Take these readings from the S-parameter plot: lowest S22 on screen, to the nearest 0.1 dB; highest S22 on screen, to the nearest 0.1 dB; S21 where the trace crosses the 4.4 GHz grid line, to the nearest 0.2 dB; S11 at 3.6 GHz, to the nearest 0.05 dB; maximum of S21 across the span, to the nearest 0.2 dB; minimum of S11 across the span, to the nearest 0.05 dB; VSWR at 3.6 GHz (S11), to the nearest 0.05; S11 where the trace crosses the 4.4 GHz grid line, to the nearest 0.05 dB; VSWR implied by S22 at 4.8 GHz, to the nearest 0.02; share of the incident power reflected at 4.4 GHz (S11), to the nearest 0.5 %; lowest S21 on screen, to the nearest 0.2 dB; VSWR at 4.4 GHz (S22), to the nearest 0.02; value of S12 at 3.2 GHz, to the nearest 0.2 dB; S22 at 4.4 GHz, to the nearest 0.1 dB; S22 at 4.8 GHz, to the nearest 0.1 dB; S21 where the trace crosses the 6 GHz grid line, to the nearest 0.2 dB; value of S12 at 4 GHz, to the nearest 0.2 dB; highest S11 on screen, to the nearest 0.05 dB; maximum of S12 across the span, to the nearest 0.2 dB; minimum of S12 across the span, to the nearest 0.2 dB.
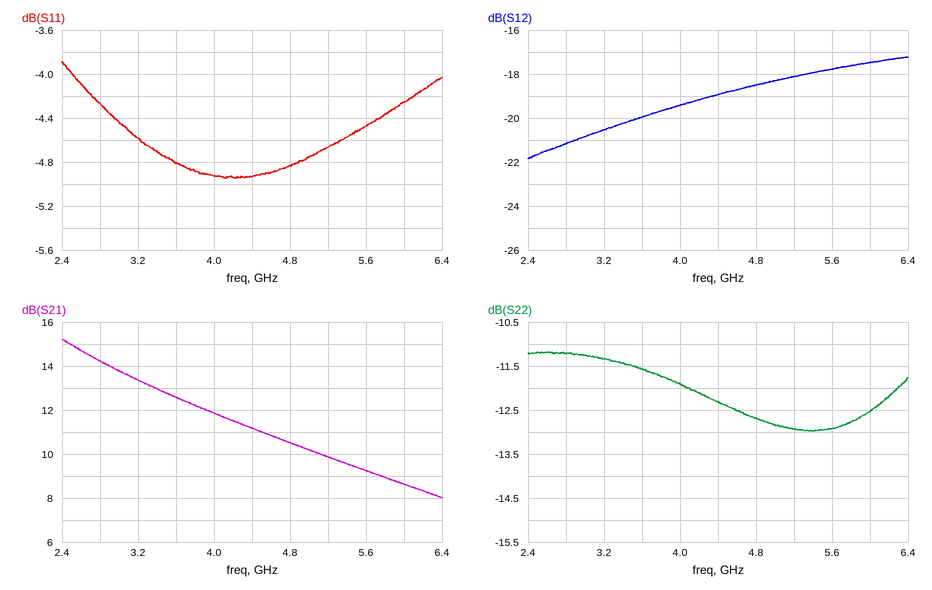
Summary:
-13.0 dB
-11.2 dB
11.2 dB
-4.80 dB
15.2 dB
-4.95 dB
3.70
-4.95 dB
1.60
32.0 %
8.0 dB
1.64
-20.6 dB
-12.3 dB
-12.7 dB
8.6 dB
-19.4 dB
-3.90 dB
-17.2 dB
-21.8 dB
